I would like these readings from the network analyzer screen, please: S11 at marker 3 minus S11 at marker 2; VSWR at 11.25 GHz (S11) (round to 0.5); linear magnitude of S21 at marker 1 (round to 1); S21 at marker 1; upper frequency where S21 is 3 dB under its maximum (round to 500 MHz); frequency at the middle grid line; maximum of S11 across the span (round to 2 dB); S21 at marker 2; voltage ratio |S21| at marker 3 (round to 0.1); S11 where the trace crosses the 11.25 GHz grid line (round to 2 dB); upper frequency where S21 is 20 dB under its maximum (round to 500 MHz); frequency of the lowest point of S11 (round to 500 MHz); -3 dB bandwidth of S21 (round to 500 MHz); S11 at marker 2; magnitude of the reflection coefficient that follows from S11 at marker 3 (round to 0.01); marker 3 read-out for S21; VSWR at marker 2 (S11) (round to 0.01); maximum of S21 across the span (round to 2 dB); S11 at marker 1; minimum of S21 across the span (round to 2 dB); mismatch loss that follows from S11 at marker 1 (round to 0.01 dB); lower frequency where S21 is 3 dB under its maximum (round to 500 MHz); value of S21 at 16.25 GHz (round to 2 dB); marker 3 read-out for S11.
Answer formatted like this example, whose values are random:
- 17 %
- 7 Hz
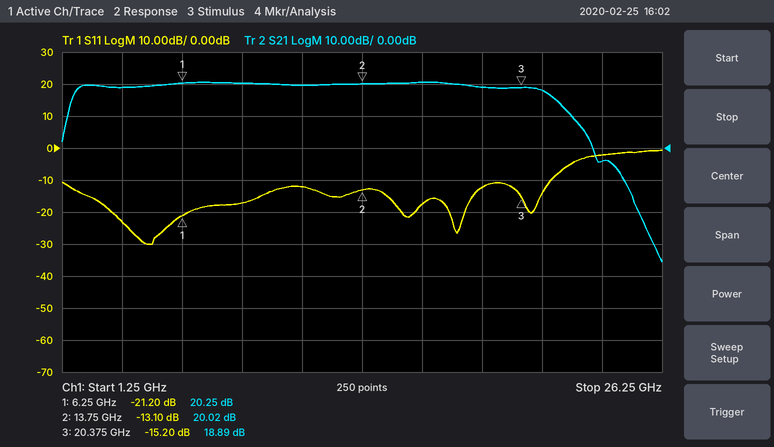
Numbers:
- -2.10 dB
- 1.5
- 10
- 20.25 dB
- 21.5 GHz
- 13.75 GHz
- 0 dB
- 20.02 dB
- 8.8
- -12 dB
- 23.5 GHz
- 5.0 GHz
- 19.5 GHz
- -13.10 dB
- 0.17
- 18.89 dB
- 1.57
- 20 dB
- -21.20 dB
- -36 dB
- 0.03 dB
- 2.0 GHz
- 20 dB
- -15.20 dB
